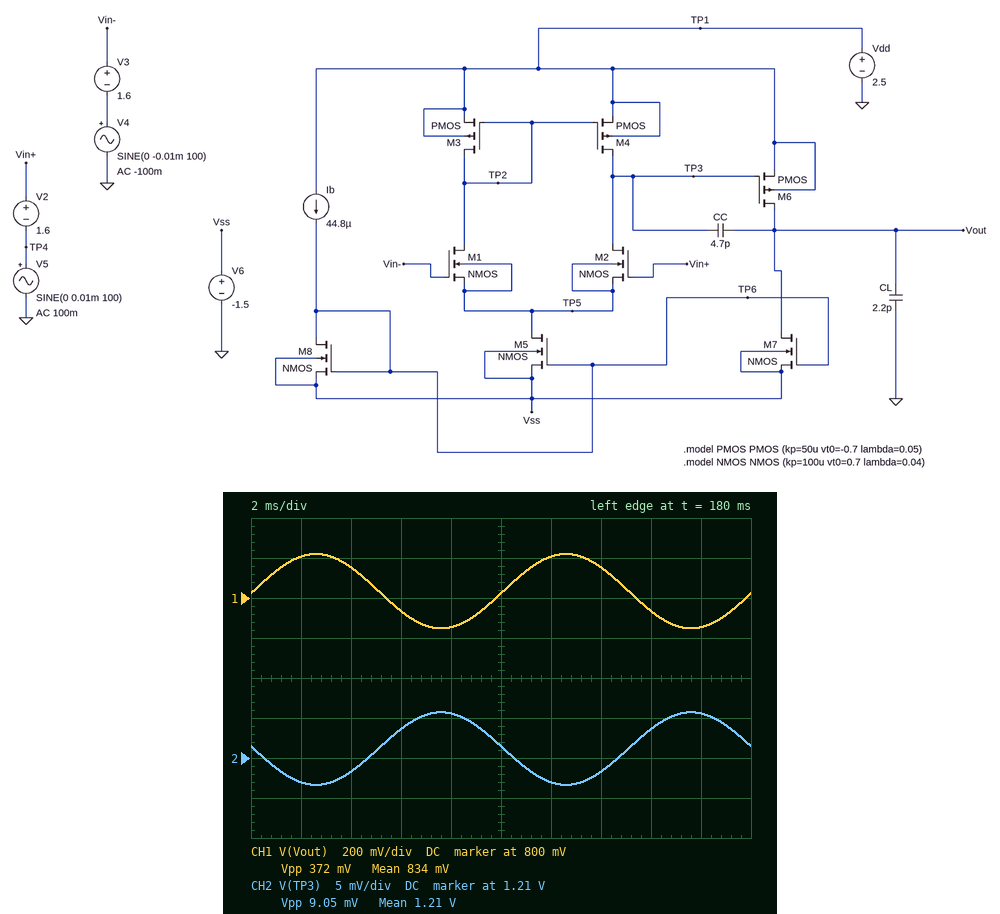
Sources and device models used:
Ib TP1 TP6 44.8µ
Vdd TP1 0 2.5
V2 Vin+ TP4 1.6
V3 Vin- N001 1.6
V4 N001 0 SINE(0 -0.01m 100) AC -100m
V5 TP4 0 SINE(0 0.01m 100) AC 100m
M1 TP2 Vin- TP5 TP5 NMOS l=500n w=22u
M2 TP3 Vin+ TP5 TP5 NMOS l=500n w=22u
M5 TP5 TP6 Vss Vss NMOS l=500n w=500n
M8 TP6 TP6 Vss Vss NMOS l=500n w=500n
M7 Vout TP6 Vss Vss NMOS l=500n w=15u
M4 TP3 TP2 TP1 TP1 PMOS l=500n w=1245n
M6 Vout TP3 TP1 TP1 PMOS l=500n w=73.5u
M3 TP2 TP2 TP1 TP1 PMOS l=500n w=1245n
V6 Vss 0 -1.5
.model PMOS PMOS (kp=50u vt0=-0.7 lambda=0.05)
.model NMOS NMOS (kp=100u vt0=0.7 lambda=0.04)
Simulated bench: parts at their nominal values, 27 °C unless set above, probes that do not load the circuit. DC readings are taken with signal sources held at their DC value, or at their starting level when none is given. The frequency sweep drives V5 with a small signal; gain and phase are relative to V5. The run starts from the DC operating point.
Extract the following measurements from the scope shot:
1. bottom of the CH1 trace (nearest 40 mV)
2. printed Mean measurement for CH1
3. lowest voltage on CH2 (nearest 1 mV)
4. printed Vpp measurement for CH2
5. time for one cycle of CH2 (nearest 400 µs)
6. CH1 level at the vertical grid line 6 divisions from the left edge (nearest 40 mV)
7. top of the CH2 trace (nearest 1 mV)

640 mV
834 mV
1.207 V
9.05 mV
10.0 ms
1.00 V
1.216 V
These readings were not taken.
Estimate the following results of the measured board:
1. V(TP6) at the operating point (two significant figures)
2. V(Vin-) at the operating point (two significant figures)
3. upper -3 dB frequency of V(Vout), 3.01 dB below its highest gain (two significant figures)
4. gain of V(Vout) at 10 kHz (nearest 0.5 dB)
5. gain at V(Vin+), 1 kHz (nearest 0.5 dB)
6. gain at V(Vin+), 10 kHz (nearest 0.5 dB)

120 mV
1.6 V
1.6 kHz
64.0 dB
0 dB
0 dB
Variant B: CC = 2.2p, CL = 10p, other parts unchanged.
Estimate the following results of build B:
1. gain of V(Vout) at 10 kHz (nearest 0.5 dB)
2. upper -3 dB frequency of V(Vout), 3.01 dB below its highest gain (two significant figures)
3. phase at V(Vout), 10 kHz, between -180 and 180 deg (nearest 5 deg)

70.5 dB
3.4 kHz
-70 deg
